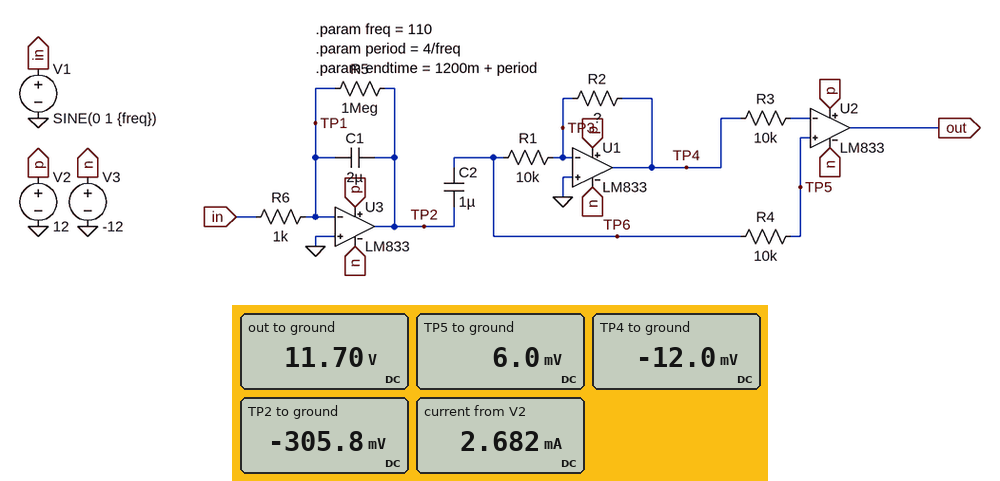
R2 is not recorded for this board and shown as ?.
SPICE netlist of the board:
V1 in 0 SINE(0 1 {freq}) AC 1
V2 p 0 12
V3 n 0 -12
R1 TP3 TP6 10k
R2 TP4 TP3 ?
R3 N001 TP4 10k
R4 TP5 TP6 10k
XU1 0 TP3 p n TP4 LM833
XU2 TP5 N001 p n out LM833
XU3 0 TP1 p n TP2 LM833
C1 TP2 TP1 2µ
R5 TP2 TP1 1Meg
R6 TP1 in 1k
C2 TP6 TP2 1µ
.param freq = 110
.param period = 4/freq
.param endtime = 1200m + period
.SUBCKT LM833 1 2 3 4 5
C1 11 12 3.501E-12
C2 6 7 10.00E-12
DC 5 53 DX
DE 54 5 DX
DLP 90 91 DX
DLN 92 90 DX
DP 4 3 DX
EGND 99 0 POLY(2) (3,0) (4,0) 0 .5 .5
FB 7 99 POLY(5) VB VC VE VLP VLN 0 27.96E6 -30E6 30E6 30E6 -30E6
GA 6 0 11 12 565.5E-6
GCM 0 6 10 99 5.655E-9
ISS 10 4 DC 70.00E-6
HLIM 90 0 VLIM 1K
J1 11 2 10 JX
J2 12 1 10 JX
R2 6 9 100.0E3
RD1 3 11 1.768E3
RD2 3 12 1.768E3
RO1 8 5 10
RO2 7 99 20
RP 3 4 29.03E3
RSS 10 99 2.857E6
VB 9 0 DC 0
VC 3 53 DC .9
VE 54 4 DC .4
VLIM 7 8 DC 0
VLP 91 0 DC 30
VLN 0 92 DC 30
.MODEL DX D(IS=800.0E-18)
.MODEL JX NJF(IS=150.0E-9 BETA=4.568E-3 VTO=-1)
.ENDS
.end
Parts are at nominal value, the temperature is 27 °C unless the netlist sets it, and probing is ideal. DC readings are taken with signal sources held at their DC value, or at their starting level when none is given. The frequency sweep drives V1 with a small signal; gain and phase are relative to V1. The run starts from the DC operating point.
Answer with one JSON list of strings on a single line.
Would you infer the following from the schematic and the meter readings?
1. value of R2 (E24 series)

["20 kΩ"]
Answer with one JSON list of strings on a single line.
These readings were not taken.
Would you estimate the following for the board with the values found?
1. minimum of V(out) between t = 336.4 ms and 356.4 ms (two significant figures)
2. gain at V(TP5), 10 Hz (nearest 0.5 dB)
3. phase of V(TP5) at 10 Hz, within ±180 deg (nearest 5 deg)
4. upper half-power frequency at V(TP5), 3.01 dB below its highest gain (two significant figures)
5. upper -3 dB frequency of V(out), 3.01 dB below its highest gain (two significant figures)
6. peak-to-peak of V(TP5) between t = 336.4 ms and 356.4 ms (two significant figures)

["-12 V", "12.5 dB", "150 deg", "16 Hz", "16 Hz", "1.4 V"]
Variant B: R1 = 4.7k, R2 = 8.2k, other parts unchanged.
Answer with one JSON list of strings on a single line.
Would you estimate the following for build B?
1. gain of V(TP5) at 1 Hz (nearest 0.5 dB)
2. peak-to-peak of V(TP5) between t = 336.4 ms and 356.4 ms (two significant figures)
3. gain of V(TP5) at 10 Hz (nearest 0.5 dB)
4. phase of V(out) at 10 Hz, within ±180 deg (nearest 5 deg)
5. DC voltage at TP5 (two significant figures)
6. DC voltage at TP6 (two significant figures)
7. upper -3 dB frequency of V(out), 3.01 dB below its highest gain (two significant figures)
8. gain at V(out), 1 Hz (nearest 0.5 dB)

["7.5 dB", "1.4 V", "7.0 dB", "165 deg", "4.4 mV", "1.4 mV", "34 Hz", "28.5 dB"]
